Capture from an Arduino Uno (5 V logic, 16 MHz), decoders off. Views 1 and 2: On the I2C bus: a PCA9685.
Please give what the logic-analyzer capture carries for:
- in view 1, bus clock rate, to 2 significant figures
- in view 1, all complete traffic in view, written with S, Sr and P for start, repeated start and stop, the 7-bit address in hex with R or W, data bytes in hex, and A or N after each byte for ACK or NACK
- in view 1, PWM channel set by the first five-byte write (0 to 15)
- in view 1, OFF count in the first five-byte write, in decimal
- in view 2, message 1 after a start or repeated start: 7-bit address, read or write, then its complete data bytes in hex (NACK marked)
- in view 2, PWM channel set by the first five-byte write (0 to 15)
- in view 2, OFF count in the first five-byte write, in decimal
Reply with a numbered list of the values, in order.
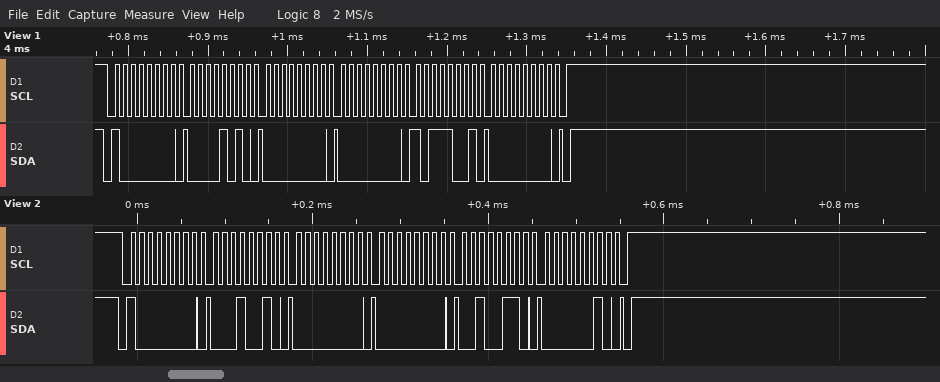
1. 100 kHz
2. S 40W A 0A A 00 A 00 A B9 A 00 A P
3. 1
4. 185
5. 0x40 write: 12 00 00 26 02
6. 3
7. 550
